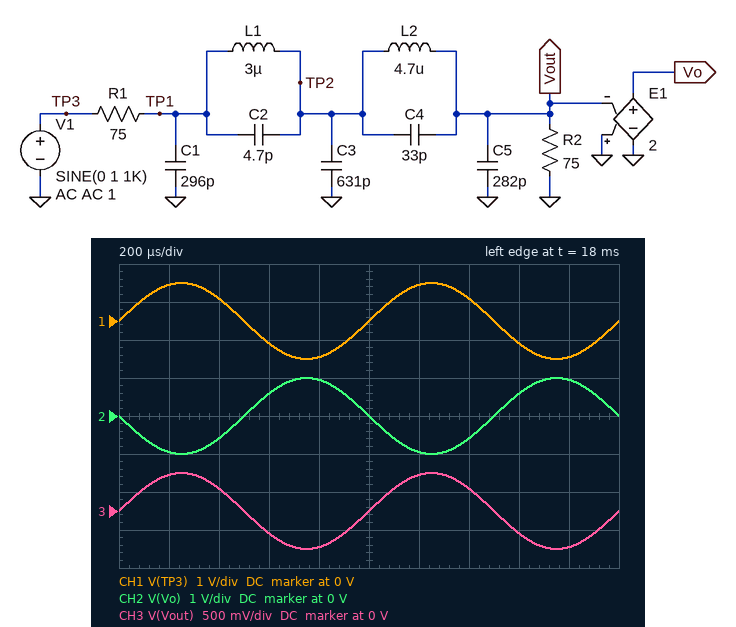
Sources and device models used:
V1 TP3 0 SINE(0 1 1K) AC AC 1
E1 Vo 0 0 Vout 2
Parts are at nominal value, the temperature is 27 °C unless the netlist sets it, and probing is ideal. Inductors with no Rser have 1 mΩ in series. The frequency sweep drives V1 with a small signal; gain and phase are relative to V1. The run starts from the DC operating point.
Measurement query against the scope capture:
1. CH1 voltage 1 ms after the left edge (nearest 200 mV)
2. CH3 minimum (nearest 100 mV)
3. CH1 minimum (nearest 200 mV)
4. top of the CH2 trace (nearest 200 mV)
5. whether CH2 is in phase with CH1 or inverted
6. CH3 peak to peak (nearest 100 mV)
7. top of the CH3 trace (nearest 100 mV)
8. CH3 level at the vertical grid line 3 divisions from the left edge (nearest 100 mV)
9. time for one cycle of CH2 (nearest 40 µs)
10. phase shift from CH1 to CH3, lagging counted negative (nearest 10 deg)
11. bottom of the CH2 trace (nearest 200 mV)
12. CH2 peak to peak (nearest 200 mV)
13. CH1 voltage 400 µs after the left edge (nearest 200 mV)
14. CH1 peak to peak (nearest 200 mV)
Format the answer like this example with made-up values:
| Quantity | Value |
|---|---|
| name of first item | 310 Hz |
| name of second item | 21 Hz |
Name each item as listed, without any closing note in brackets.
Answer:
| Quantity | Value |
|---|---|
| CH1 voltage 1 ms after the left edge | 0 V |
| CH3 minimum | -500 mV |
| CH1 minimum | -1.0 V |
| top of the CH2 trace | 1.0 V |
| whether CH2 is in phase with CH1 or inverted | inverted |
| CH3 peak to peak | 1.0 V |
| top of the CH3 trace | 500 mV |
| CH3 level at the vertical grid line 3 divisions from the left edge | -300 mV |
| time for one cycle of CH2 | 1.00 ms |
| phase shift from CH1 to CH3, lagging counted negative | 0 deg |
| bottom of the CH2 trace | -1.0 V |
| CH2 peak to peak | 2.0 V |
| CH1 voltage 400 µs after the left edge | 600 mV |
| CH1 peak to peak | 2.0 V |
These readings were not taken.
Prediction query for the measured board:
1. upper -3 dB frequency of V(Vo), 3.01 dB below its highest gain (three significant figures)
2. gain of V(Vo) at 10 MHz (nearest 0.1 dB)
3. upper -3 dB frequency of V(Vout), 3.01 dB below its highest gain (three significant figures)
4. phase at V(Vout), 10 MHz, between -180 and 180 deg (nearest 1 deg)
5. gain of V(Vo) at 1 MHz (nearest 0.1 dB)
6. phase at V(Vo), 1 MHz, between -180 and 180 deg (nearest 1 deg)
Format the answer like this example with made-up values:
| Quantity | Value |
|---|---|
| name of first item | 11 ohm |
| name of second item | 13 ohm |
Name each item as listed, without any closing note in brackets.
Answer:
| Quantity | Value |
|---|---|
| upper -3 dB frequency of V(Vo), 3.01 dB below its highest gain | 5.29 MHz |
| gain of V(Vo) at 10 MHz | -37.4 dB |
| upper -3 dB frequency of V(Vout), 3.01 dB below its highest gain | 5.29 MHz |
| phase at V(Vout), 10 MHz, between -180 and 180 deg | -5 deg |
| gain of V(Vo) at 1 MHz | 0 dB |
| phase at V(Vo), 1 MHz, between -180 and 180 deg | 145 deg |
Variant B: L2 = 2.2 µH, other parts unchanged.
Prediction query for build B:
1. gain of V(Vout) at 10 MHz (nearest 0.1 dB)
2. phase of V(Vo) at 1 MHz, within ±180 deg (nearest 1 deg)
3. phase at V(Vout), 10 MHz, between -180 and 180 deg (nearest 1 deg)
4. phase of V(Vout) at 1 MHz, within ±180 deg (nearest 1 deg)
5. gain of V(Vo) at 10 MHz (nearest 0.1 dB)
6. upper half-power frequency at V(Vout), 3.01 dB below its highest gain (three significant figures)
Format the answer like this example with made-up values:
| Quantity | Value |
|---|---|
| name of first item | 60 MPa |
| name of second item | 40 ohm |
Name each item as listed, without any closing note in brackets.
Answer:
| Quantity | Value |
|---|---|
| gain of V(Vout) at 10 MHz | -28.9 dB |
| phase of V(Vo) at 1 MHz, within ±180 deg | 151 deg |
| phase at V(Vout), 10 MHz, between -180 and 180 deg | 5 deg |
| phase of V(Vout) at 1 MHz, within ±180 deg | -29 deg |
| gain of V(Vo) at 10 MHz | -22.9 dB |
| upper half-power frequency at V(Vout), 3.01 dB below its highest gain | 6.99 MHz |
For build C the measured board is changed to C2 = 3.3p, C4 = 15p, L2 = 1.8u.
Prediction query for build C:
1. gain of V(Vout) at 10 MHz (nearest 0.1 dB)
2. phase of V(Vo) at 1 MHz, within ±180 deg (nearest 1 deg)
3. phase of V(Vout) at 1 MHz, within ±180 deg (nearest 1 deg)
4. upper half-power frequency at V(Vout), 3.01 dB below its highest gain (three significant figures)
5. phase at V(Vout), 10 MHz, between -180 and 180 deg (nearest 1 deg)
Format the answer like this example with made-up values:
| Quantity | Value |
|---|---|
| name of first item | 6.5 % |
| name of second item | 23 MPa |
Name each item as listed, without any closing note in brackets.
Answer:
| Quantity | Value |
|---|---|
| gain of V(Vout) at 10 MHz | -22.9 dB |
| phase of V(Vo) at 1 MHz, within ±180 deg | 152 deg |
| phase of V(Vout) at 1 MHz, within ±180 deg | -28 deg |
| upper half-power frequency at V(Vout), 3.01 dB below its highest gain | 7.40 MHz |
| phase at V(Vout), 10 MHz, between -180 and 180 deg | 18 deg |
